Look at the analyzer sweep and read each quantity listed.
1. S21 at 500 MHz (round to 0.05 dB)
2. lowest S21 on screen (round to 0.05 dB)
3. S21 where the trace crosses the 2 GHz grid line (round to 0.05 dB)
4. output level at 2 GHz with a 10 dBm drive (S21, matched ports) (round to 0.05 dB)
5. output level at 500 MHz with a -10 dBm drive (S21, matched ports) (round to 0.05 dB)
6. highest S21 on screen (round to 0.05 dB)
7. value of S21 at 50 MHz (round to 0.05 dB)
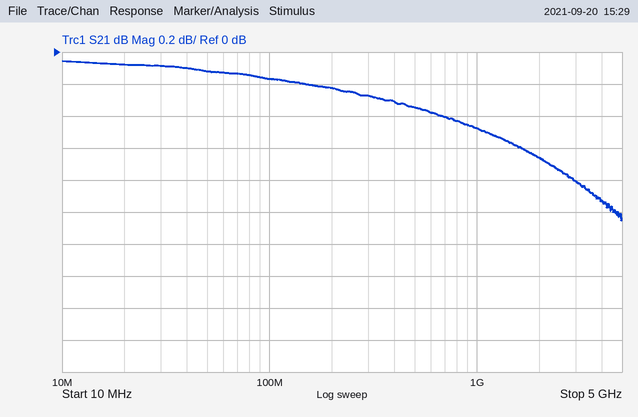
-0.35 dB
-1.05 dB
-0.65 dB
9.35 dBm
-10.35 dBm
-0.05 dB
-0.10 dB
